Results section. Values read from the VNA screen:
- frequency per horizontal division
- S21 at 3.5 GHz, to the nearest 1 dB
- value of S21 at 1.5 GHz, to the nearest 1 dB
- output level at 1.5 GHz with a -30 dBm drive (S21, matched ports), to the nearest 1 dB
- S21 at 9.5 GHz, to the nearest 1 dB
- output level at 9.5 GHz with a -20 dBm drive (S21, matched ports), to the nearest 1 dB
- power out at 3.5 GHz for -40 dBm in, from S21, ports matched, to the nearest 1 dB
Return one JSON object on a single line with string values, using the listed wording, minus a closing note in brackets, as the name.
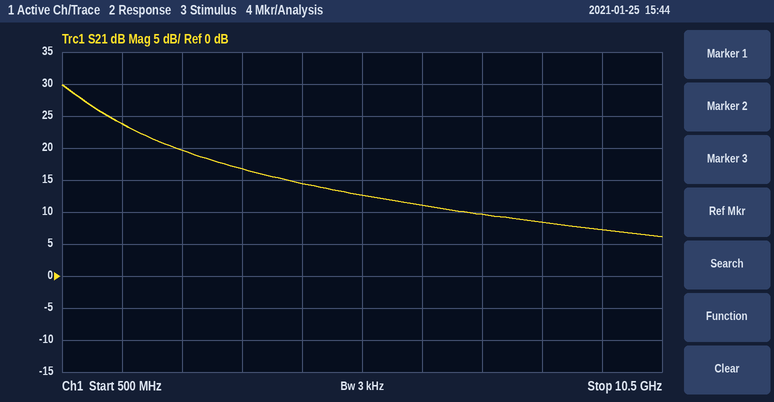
{"frequency per horizontal division": "1 GHz", "S21 at 3.5 GHz, to the nearest 1 dB": "17 dB", "value of S21 at 1.5 GHz, to the nearest 1 dB": "24 dB", "output level at 1.5 GHz with a -30 dBm drive (S21, matched ports), to the nearest 1 dB": "-6 dBm", "S21 at 9.5 GHz, to the nearest 1 dB": "7 dB", "output level at 9.5 GHz with a -20 dBm drive (S21, matched ports), to the nearest 1 dB": "-13 dBm", "power out at 3.5 GHz for -40 dBm in, from S21, ports matched, to the nearest 1 dB": "-23 dBm"}
